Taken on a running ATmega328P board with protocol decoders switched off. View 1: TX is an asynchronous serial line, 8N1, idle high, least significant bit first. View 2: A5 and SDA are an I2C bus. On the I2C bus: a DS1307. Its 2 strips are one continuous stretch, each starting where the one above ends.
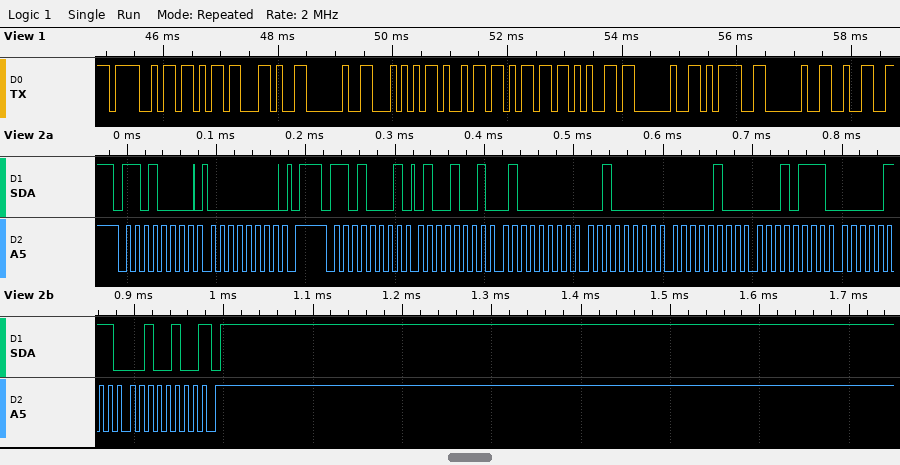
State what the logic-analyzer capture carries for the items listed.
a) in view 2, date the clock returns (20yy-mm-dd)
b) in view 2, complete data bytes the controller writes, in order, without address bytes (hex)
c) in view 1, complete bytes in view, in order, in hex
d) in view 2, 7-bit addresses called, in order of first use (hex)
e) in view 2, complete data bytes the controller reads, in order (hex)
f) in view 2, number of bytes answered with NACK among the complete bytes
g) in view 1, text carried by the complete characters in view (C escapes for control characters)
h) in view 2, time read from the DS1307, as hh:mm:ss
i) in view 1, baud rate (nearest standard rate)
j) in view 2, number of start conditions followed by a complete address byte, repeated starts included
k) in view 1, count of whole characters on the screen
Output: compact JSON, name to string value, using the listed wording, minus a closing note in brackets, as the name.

{"in view 2, date the clock returns": "2024-07-17", "in view 2, complete data bytes the controller writes, in order, without address bytes": "00", "in view 1, complete bytes in view, in order, in hex": "4F 6B 2C 20 54 69 6D 65 20 3D 20 32", "in view 2, 7-bit addresses called, in order of first use": "0x68", "in view 2, complete data bytes the controller reads, in order": "49 40 20 04 17 07 24", "in view 2, number of bytes answered with NACK among the complete bytes": "1", "in view 1, text carried by the complete characters in view": "\"Ok, Time = 2\"", "in view 2, time read from the DS1307, as hh:mm:ss": "20:40:49", "in view 1, baud rate": "9600 baud", "in view 2, number of start conditions followed by a complete address byte, repeated starts included": "2", "in view 1, count of whole characters on the screen": "12"}
